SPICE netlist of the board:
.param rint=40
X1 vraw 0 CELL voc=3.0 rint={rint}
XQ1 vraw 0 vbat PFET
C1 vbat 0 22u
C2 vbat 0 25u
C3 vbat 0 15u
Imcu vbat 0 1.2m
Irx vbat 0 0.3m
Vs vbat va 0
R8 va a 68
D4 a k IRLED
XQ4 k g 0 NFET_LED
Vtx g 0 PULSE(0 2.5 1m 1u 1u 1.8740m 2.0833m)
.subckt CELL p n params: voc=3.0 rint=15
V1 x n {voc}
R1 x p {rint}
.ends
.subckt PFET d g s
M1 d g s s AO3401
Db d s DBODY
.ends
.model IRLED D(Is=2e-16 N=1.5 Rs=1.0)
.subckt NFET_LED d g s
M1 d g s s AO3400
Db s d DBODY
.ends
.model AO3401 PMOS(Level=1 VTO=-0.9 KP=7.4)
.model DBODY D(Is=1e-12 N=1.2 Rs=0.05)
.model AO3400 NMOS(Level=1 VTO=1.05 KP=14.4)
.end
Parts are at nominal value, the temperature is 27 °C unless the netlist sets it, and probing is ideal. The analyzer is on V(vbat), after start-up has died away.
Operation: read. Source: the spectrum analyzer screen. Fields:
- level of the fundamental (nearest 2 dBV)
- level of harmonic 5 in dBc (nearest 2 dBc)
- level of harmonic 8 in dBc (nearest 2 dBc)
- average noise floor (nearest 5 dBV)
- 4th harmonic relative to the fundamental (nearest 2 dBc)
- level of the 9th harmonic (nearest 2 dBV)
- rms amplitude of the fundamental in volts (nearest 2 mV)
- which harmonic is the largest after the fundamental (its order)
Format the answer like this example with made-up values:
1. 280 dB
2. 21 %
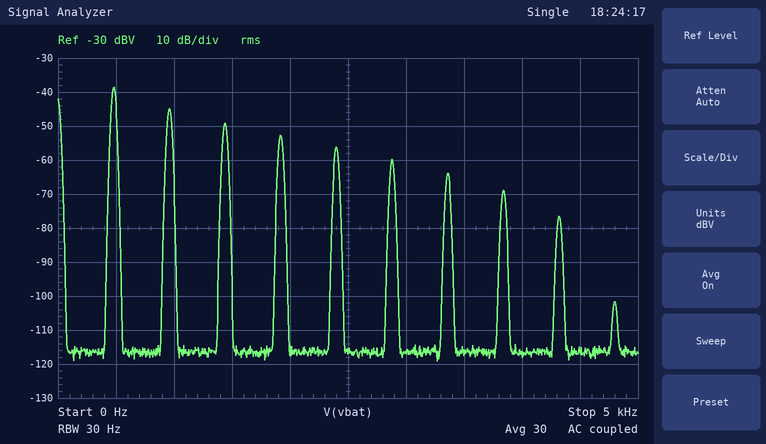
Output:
1. -38 dBV
2. -18 dBc
3. -30 dBc
4. -115 dBV
5. -14 dBc
6. -76 dBV
7. 12 mV
8. 2
